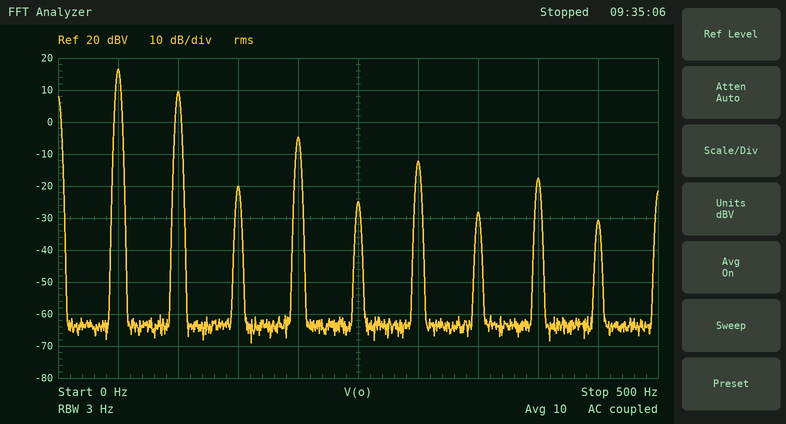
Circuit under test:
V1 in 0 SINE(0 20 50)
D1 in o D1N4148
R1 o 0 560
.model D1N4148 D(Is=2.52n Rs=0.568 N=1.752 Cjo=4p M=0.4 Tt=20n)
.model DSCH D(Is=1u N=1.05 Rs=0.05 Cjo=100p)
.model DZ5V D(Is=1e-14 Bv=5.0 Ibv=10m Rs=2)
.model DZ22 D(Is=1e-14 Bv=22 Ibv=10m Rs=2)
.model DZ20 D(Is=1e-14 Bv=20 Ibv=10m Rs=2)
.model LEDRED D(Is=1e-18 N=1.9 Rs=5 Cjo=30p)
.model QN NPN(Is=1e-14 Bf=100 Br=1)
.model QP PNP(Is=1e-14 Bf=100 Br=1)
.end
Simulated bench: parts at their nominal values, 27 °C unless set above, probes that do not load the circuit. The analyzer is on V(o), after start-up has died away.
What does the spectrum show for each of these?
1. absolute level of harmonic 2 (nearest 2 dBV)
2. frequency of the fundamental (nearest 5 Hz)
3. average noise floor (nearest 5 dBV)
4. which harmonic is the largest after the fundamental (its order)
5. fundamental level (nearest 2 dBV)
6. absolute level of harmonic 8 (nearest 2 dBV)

10 dBV
50 Hz
-65 dBV
2
16 dBV
-18 dBV
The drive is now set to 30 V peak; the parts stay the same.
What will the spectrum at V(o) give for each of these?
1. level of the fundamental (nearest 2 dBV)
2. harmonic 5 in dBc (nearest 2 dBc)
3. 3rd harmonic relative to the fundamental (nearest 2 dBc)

20 dBV
-44 dBc
-40 dBc
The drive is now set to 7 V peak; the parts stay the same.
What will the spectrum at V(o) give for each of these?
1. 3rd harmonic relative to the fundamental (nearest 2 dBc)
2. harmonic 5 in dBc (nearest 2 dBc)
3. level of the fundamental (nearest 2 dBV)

-28 dBc
-32 dBc
6 dBV
